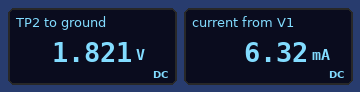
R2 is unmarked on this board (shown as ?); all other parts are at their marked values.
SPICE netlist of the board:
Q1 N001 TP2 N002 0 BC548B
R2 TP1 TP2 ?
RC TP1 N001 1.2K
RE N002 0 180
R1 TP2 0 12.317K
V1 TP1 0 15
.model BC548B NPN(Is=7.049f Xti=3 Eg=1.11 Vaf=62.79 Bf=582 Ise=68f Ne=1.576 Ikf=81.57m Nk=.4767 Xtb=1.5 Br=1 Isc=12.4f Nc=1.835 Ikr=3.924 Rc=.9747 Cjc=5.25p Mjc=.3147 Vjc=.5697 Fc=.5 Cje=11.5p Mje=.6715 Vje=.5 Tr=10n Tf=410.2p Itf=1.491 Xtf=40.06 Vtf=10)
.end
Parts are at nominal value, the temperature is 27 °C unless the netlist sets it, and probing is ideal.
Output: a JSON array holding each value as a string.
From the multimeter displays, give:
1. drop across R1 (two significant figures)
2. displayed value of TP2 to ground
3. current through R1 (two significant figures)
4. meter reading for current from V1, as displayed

["1.8 V", "1.821 V", "150 µA", "6.32 mA"]
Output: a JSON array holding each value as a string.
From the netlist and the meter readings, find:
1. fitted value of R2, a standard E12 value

["82 kΩ"]
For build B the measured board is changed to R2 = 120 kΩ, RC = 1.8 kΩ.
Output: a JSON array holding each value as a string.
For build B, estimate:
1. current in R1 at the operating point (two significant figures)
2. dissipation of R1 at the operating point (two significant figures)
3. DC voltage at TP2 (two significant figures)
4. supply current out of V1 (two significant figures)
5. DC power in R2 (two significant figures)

["110 µA", "140 µW", "1.3 V", "3.6 mA", "1.6 mW"]
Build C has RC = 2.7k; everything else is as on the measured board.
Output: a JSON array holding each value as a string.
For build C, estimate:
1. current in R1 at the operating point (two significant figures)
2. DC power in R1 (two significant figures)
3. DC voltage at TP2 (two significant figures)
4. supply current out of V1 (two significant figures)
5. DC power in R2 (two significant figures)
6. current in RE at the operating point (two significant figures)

["130 µA", "220 µW", "1.6 V", "5.3 mA", "2.2 mW", "5.2 mA"]
